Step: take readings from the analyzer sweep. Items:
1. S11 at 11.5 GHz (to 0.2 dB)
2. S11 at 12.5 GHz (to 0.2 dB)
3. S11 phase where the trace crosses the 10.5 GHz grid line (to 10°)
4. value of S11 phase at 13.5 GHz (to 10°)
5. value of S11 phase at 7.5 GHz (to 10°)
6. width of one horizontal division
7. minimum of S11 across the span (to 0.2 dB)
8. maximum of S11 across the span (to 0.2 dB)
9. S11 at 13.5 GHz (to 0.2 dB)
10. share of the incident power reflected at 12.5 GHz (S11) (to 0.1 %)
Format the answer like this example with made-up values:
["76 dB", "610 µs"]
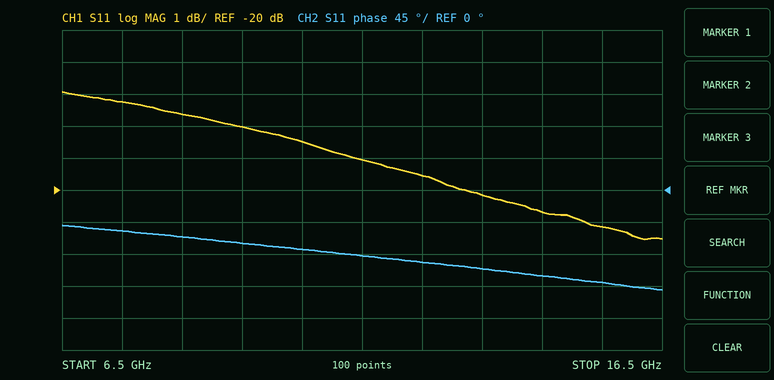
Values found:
["-19.0 dB", "-19.6 dB", "-80°", "-110°", "-60°", "1 GHz", "-21.6 dB", "-17.0 dB", "-20.2 dB", "1.1 %"]
